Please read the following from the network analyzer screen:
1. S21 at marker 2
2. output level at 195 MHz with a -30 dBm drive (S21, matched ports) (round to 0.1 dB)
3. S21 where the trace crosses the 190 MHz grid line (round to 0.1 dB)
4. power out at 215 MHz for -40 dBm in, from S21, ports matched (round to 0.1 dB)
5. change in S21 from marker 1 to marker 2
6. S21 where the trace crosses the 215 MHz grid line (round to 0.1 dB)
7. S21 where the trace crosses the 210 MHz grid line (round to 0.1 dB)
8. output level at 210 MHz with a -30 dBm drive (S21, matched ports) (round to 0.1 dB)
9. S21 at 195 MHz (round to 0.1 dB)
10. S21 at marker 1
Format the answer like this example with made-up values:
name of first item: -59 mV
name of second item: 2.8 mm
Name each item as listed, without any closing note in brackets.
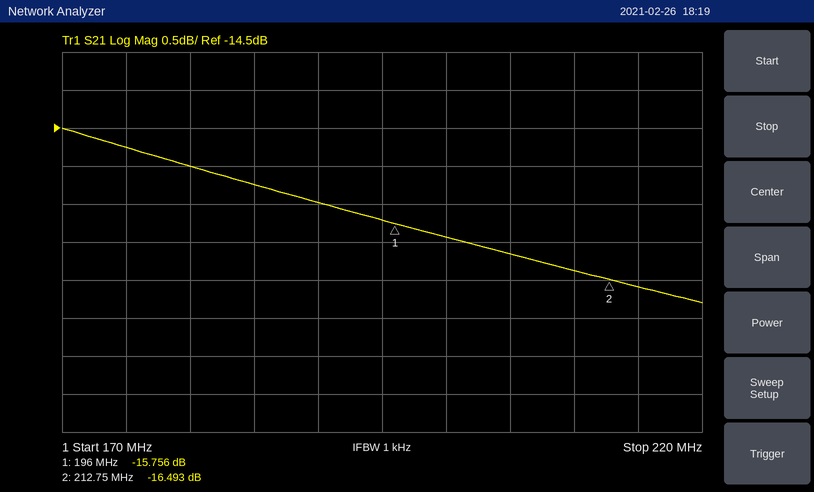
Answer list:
S21 at marker 2: -16.493 dB
output level at 195 MHz with a -30 dBm drive (S21, matched ports): -45.7 dBm
S21 where the trace crosses the 190 MHz grid line: -15.5 dB
power out at 215 MHz for -40 dBm in, from S21, ports matched: -56.6 dBm
change in S21 from marker 1 to marker 2: -0.737 dB
S21 where the trace crosses the 215 MHz grid line: -16.6 dB
S21 where the trace crosses the 210 MHz grid line: -16.4 dB
output level at 210 MHz with a -30 dBm drive (S21, matched ports): -46.4 dBm
S21 at 195 MHz: -15.7 dB
S21 at marker 1: -15.756 dB
